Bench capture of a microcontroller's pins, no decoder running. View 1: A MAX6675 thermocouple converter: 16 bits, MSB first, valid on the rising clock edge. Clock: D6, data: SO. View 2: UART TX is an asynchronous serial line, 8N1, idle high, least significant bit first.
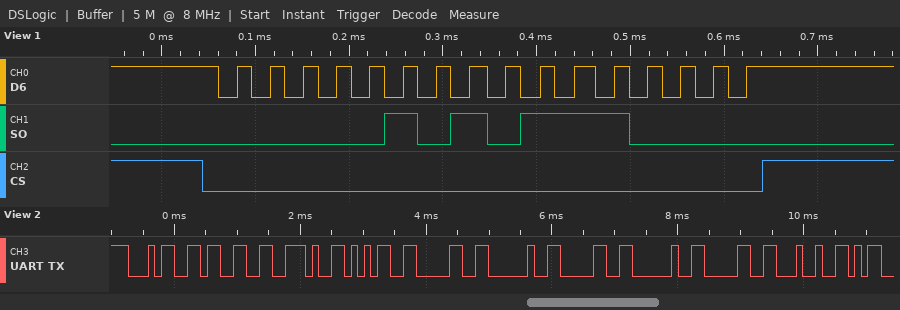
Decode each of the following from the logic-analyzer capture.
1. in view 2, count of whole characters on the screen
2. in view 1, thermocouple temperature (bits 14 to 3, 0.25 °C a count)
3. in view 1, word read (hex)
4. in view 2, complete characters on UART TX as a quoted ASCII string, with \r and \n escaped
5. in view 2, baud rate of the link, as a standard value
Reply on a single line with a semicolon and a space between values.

10; 43.50 °C; 0x0570; "43.50 0 0$"; 9600 baud
